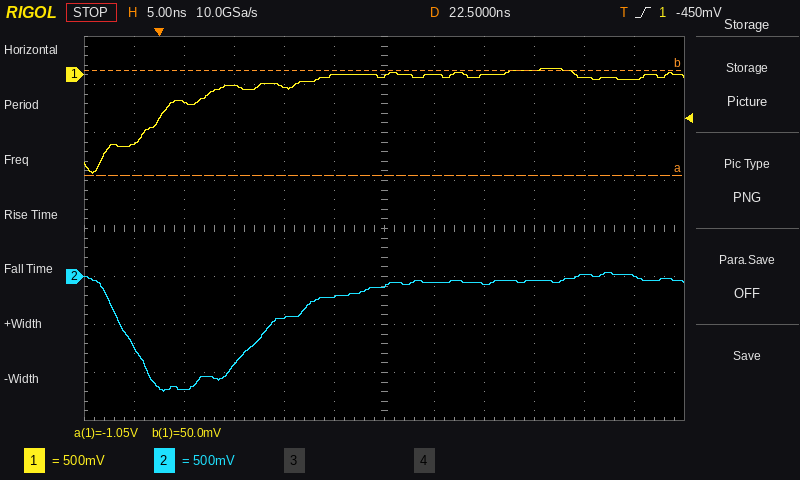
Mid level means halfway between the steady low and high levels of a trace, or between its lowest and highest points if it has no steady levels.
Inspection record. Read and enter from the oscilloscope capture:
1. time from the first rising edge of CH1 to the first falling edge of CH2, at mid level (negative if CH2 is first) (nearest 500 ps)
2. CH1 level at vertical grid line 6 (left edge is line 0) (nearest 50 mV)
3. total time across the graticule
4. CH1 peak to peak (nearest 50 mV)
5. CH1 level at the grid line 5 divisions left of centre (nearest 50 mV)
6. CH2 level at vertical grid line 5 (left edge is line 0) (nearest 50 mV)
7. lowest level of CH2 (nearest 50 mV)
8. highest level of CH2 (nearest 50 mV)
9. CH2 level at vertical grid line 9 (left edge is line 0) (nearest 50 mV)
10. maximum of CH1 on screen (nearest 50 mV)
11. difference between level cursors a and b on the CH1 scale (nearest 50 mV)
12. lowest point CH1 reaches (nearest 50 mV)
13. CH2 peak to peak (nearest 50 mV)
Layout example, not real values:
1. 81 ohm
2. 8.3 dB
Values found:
1. -3.5 ns
2. 0 mV
3. 60 ns
4. 1.10 V
5. -700 mV
6. -200 mV
7. -1.20 V
8. 50 mV
9. -50 mV
10. 50 mV
11. 1.10 V
12. -1.05 V
13. 1.25 V
